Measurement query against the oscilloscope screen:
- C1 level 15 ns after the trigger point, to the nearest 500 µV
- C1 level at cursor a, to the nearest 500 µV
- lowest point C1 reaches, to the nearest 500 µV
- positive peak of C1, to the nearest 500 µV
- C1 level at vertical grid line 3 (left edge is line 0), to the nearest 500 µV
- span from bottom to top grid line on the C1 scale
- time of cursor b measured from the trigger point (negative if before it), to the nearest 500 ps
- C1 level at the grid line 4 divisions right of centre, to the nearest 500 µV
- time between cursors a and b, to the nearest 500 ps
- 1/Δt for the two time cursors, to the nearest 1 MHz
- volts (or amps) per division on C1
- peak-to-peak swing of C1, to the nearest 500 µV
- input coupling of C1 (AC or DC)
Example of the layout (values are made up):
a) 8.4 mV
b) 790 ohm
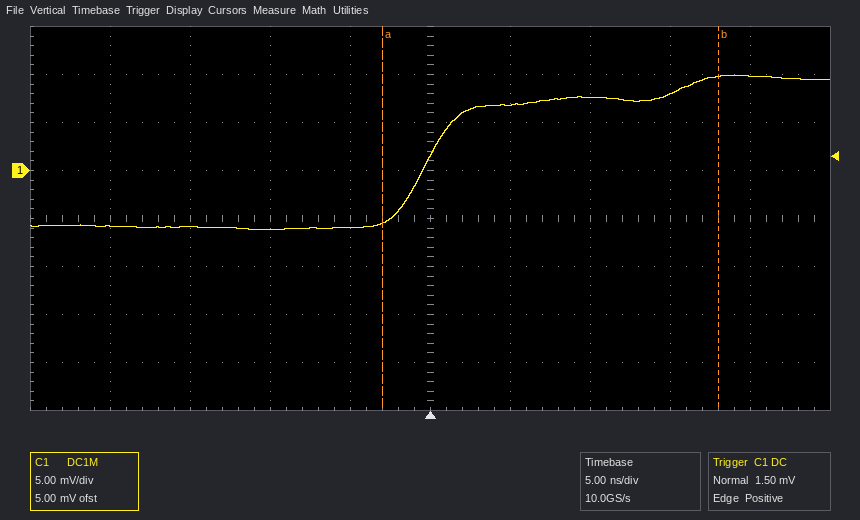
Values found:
a) 8.0 mV
b) -5.5 mV
c) -6.0 mV
d) 10.0 mV
e) -6.0 mV
f) 40 mV
g) +18.0 ns
h) 10.0 mV
i) 21.0 ns
j) 48 MHz
k) 5 mV
l) 16.0 mV
m) DC
